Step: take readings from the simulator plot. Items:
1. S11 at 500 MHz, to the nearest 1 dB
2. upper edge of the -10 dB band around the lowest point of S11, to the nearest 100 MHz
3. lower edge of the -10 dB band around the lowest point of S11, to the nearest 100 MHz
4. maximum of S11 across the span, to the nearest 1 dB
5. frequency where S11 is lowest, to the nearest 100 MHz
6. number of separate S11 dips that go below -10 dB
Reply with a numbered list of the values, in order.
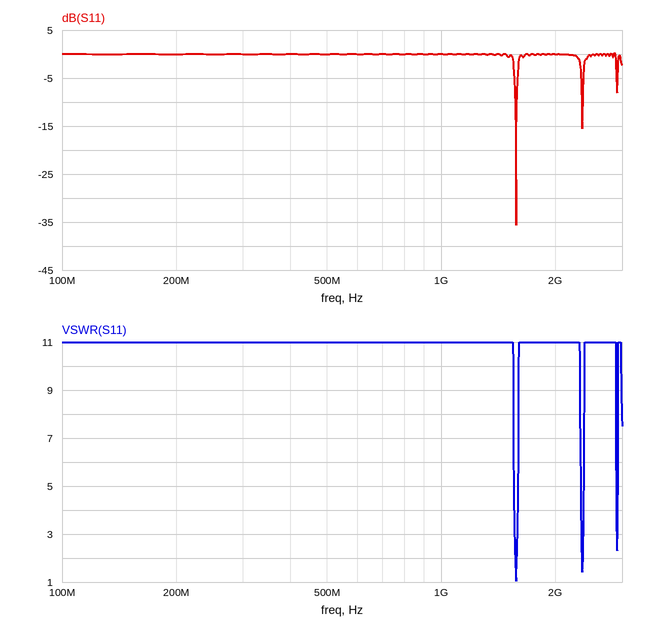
1. 0 dB
2. 1.6 GHz
3. 1.6 GHz
4. 0 dB
5. 1.6 GHz
6. 2
